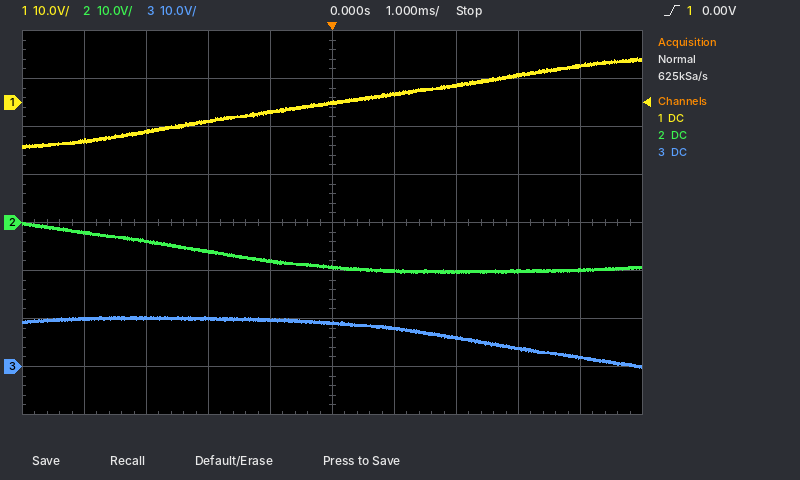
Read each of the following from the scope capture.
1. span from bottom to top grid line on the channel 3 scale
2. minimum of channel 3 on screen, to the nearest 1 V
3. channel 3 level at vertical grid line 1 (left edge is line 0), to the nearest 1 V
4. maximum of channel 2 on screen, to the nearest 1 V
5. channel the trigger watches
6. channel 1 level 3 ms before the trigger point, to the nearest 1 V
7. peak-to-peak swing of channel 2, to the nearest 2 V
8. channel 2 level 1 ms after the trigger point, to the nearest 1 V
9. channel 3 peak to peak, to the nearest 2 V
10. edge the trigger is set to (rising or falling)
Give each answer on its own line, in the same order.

80 V
0 V
10 V
0 V
channel 1
-6 V
10 V
-10 V
10 V
rising
